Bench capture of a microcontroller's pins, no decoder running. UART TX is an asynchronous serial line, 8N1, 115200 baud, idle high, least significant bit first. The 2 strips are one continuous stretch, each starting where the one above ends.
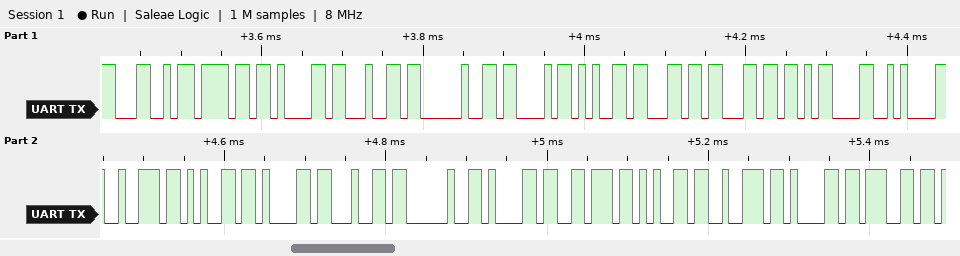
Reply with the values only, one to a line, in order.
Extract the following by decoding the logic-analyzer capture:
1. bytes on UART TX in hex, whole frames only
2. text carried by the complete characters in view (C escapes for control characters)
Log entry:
4C 6F 61 64 20 43 65 6C 6C 0D 0A 72 65 61 64 20 61 76 65 72 61 67
"Load Cell\r\nread averag"
